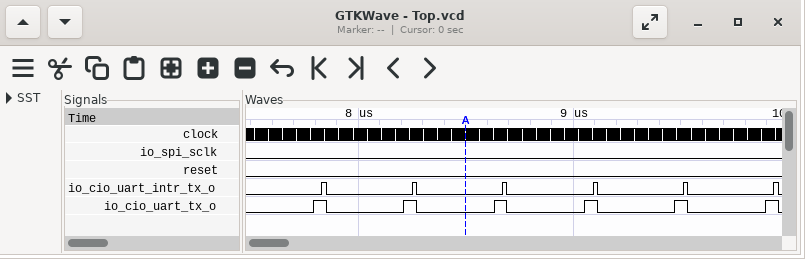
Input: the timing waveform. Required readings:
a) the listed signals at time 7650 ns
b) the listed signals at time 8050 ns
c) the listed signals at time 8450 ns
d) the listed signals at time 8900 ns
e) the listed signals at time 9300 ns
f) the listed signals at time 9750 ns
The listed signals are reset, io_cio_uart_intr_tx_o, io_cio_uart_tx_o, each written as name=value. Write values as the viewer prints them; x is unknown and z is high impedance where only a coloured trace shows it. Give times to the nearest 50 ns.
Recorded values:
reset=0, io_cio_uart_intr_tx_o=0, io_cio_uart_tx_o=0
reset=0, io_cio_uart_intr_tx_o=0, io_cio_uart_tx_o=0
reset=0, io_cio_uart_intr_tx_o=0, io_cio_uart_tx_o=0
reset=0, io_cio_uart_intr_tx_o=0, io_cio_uart_tx_o=0
reset=0, io_cio_uart_intr_tx_o=0, io_cio_uart_tx_o=0
reset=0, io_cio_uart_intr_tx_o=0, io_cio_uart_tx_o=0
